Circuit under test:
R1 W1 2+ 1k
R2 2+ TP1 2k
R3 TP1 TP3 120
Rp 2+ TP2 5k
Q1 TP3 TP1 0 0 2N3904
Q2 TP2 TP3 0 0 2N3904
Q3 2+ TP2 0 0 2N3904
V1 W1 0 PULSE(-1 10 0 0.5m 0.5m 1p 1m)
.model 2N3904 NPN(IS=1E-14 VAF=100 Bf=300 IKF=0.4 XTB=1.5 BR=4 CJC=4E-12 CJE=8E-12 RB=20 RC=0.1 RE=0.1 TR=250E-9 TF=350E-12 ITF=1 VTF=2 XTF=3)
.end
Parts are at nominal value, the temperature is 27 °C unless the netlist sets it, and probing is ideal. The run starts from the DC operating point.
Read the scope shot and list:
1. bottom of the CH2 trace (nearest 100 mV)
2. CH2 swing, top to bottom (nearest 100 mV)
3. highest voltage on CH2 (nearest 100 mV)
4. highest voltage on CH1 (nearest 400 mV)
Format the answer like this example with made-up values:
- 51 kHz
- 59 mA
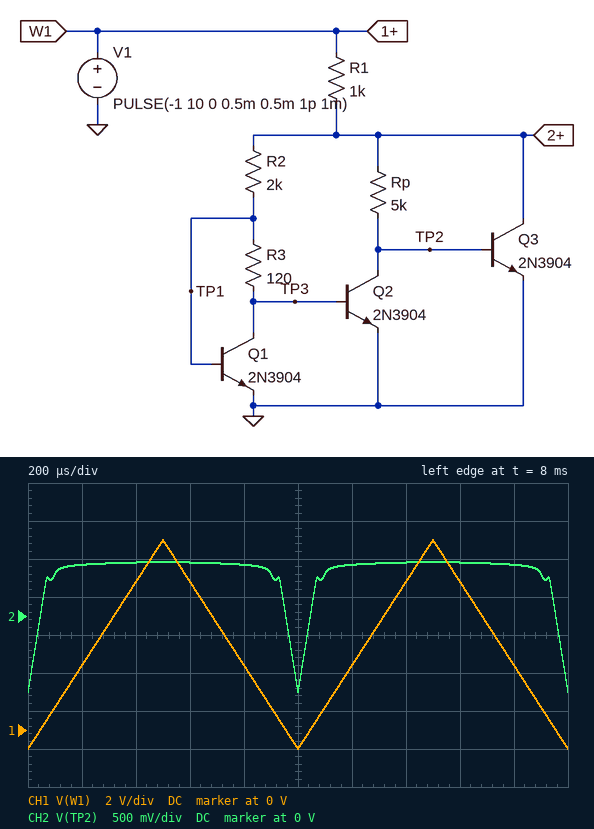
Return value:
- -1.0 V
- 1.7 V
- 700 mV
- 10.0 V
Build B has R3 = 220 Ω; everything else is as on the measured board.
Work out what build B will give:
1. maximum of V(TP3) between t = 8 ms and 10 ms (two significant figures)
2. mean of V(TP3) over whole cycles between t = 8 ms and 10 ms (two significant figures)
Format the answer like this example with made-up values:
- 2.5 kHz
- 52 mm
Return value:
- 570 mV
- 460 mV
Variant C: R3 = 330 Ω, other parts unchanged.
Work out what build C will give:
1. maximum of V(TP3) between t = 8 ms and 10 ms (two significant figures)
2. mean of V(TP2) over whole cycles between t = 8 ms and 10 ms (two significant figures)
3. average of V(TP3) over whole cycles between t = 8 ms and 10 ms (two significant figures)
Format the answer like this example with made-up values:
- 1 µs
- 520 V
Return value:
- 560 mV
- 550 mV
- 450 mV
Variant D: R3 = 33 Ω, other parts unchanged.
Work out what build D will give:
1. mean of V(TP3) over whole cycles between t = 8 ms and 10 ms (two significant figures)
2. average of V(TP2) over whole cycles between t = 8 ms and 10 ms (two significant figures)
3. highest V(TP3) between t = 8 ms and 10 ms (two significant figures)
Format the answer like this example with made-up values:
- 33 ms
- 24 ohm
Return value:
- 500 mV
- 470 mV
- 620 mV
